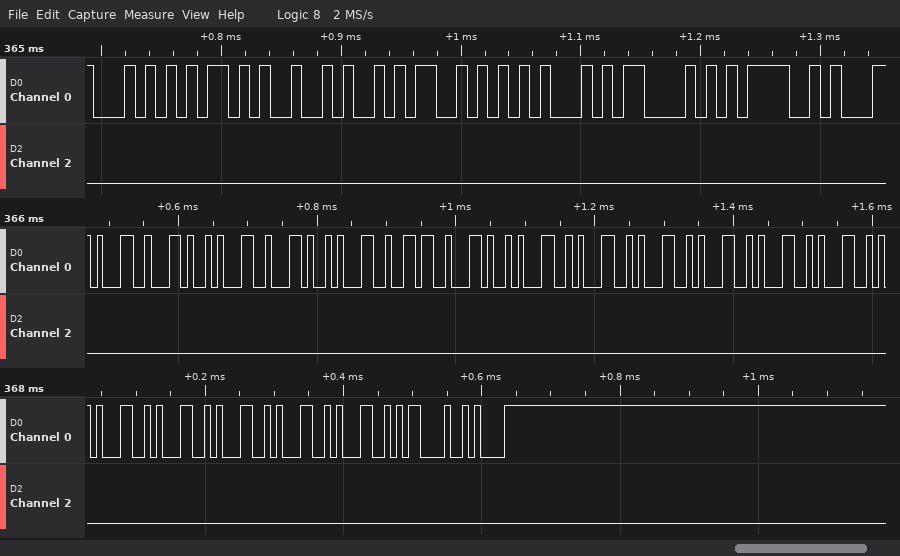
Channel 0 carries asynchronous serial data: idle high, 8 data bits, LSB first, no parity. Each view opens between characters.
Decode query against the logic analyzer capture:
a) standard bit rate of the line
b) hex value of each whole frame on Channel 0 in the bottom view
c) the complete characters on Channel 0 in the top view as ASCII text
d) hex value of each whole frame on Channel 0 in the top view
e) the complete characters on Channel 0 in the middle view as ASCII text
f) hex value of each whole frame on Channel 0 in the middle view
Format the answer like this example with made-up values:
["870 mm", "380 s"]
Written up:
["115200 baud", "31, 31, 31, 31, 31, 0D, 0A", "\"T+JSEC=\"", "54, 2B, 4A, 53, 45, 43, 3D", "\"1,1,16,111111\"", "31, 2C, 31, 2C, 31, 36, 2C, 31, 31, 31, 31, 31, 31"]
